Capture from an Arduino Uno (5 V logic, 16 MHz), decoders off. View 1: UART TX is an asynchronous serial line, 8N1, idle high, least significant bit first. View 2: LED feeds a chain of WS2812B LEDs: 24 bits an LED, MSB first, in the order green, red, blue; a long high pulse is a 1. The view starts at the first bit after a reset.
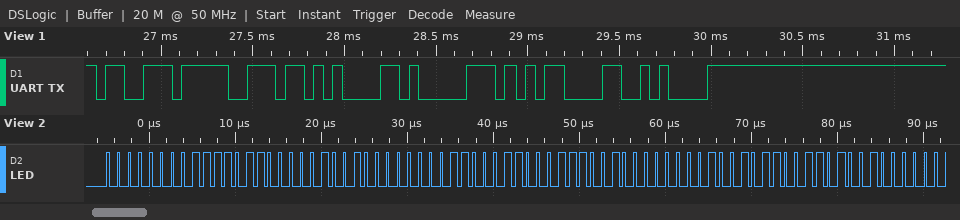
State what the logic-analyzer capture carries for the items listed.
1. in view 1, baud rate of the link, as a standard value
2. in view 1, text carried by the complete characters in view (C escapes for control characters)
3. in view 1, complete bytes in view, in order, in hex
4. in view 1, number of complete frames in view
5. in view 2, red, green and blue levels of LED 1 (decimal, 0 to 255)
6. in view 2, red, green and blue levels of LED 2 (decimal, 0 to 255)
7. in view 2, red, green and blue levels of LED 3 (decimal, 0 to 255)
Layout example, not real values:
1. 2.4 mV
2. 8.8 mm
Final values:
1. 19200 baud
2. "snap\r\n"
3. 73 6E 61 70 0D 0A
4. 6
5. 246, 0, 9
6. 198, 0, 57
7. 150, 0, 105
